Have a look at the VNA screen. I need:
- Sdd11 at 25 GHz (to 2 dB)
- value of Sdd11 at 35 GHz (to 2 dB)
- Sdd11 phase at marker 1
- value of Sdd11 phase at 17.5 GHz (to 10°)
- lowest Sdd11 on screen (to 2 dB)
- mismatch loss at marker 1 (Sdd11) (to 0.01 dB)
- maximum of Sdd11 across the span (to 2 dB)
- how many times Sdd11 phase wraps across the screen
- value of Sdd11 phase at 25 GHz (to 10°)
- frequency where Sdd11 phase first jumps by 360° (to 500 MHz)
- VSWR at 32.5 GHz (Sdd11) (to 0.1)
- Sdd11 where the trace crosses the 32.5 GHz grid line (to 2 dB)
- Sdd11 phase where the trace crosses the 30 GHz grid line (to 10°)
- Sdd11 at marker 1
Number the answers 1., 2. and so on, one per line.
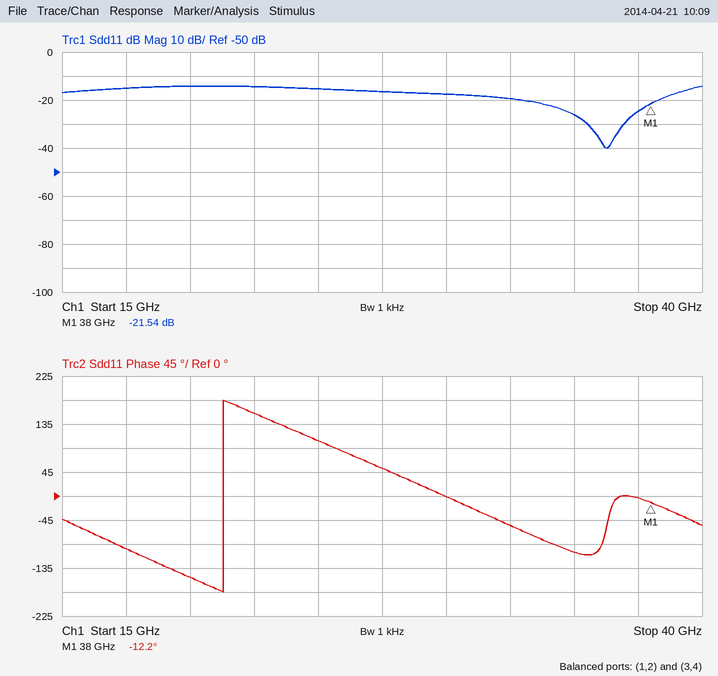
1. -16 dB
2. -26 dB
3. -12.2°
4. -100°
5. -40 dB
6. 0.03 dB
7. -14 dB
8. 1
9. 100°
10. 21.5 GHz
11. 1.2
12. -20 dB
13. 0°
14. -21.54 dB
